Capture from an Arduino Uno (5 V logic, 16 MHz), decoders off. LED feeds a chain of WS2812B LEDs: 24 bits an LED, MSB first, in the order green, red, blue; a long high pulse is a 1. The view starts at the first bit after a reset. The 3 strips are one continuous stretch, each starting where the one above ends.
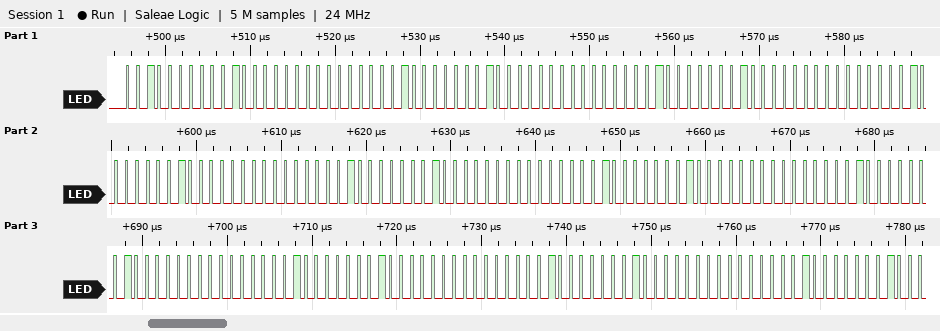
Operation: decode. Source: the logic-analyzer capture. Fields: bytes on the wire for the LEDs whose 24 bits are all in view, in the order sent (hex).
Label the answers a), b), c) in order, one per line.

a) 20 20 00 20 20 00 20 20 00 20 20 00 20 20 00 20 20 00 20 20 00 20 20 00 20 20 00
